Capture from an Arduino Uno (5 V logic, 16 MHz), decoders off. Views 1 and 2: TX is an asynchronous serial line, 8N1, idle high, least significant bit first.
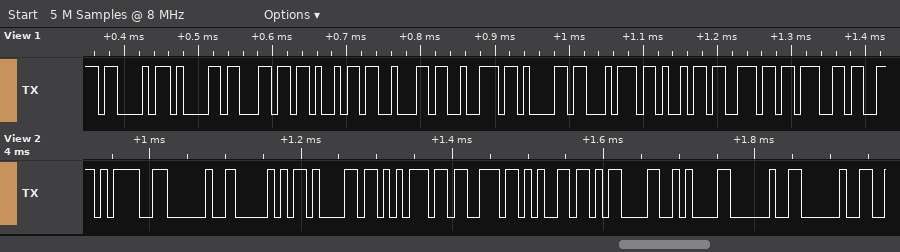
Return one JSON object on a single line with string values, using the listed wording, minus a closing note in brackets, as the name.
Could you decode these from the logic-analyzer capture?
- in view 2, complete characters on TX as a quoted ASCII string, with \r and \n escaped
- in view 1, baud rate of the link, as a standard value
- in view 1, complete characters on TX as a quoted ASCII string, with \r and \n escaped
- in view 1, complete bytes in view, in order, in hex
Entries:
{"in view 2, complete characters on TX as a quoted ASCII string, with \\r and \\n escaped": "\"= Pause\\r\\n  \"", "in view 1, baud rate of the link, as a standard value": "115200 baud", "in view 1, complete characters on TX as a quoted ASCII string, with \\r and \\n escaped": "\"Calibrating\"", "in view 1, complete bytes in view, in order, in hex": "0x43 0x61 0x6C 0x69 0x62 0x72 0x61 0x74 0x69 0x6E 0x67"}
